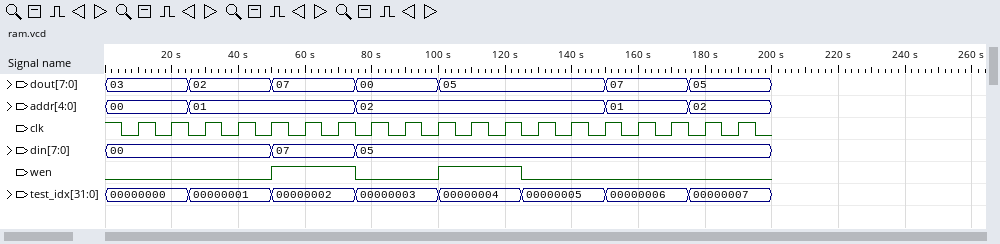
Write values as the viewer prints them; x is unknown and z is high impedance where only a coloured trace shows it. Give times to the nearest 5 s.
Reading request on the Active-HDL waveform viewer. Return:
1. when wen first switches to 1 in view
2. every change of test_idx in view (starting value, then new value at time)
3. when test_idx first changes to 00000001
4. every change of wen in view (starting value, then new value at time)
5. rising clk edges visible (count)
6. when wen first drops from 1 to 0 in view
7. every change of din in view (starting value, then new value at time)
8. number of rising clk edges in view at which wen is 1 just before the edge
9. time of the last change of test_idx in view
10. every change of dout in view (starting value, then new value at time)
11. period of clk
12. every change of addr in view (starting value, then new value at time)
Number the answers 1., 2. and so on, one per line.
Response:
1. 50 s
2. 00000000, 00000001 at 25 s, 00000002 at 50 s, 00000003 at 75 s, 00000004 at 100 s, 00000005 at 125 s, 00000006 at 150 s, 00000007 at 175 s
3. 25 s
4. 0, 1 at 50 s, 0 at 75 s, 1 at 100 s, 0 at 125 s
5. 19
6. 75 s
7. 00, 07 at 50 s, 05 at 75 s
8. 4
9. 175 s
10. 03, 02 at 25 s, 07 at 50 s, 00 at 75 s, 05 at 100 s, 07 at 150 s, 05 at 175 s
11. 10 s
12. 00, 01 at 25 s, 02 at 75 s, 01 at 150 s, 02 at 175 s
